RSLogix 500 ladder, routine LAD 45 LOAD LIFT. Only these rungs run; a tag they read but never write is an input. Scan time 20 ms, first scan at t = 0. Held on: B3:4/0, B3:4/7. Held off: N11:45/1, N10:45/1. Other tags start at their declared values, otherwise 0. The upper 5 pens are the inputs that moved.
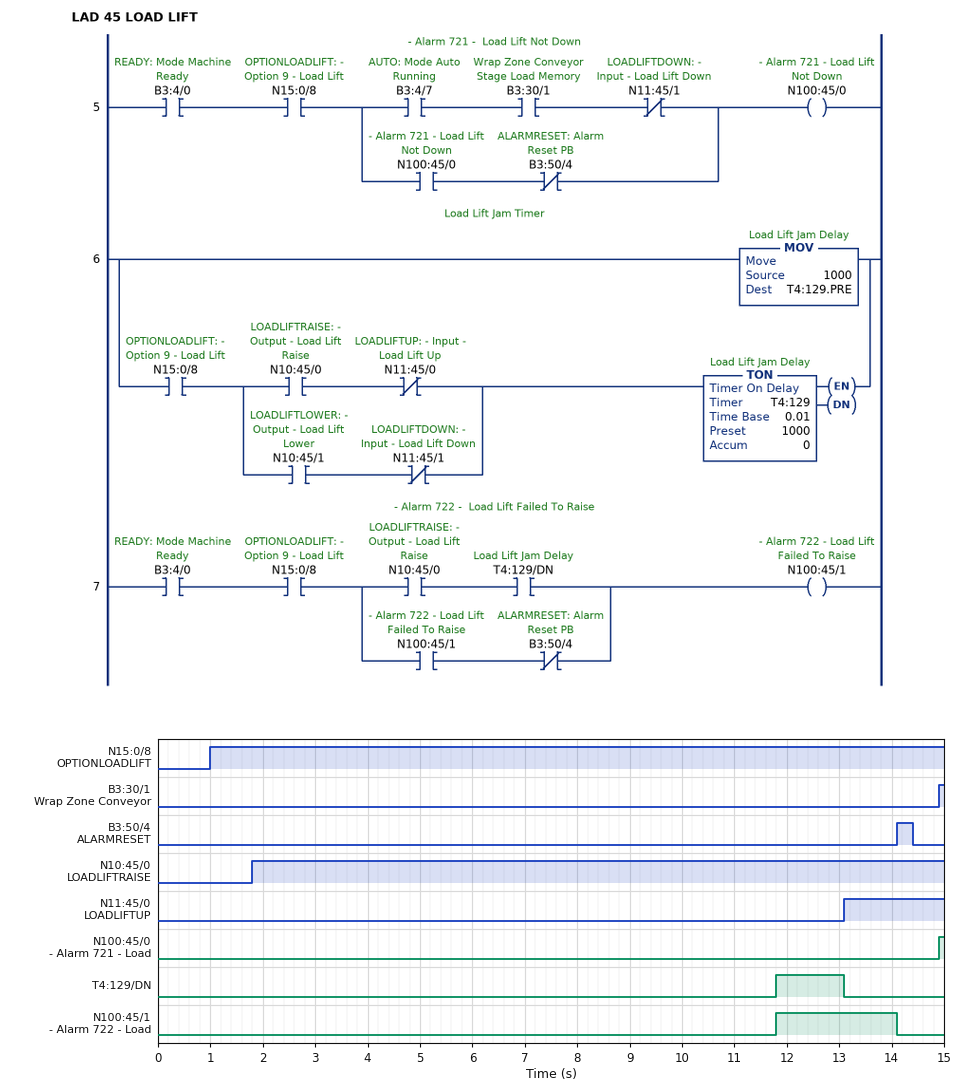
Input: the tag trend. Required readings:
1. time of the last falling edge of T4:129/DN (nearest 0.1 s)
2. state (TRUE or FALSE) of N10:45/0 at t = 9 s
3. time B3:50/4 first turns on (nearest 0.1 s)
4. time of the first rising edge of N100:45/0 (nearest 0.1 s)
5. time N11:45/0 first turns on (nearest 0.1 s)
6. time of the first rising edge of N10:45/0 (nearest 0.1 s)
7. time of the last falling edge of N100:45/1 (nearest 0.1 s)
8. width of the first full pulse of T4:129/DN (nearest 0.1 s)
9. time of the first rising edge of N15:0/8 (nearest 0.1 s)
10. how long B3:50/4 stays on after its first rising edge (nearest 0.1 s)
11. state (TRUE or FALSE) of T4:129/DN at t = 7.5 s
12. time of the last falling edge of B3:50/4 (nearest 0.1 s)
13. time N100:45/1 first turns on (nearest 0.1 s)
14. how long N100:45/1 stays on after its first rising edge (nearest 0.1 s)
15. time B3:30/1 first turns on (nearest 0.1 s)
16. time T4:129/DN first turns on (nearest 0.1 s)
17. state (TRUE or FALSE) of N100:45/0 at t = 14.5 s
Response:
13.1 s
TRUE
14.1 s
14.9 s
13.1 s
1.8 s
14.1 s
1.3 s
1.0 s
0.3 s
FALSE
14.4 s
11.8 s
2.3 s
14.9 s
11.8 s
FALSE
